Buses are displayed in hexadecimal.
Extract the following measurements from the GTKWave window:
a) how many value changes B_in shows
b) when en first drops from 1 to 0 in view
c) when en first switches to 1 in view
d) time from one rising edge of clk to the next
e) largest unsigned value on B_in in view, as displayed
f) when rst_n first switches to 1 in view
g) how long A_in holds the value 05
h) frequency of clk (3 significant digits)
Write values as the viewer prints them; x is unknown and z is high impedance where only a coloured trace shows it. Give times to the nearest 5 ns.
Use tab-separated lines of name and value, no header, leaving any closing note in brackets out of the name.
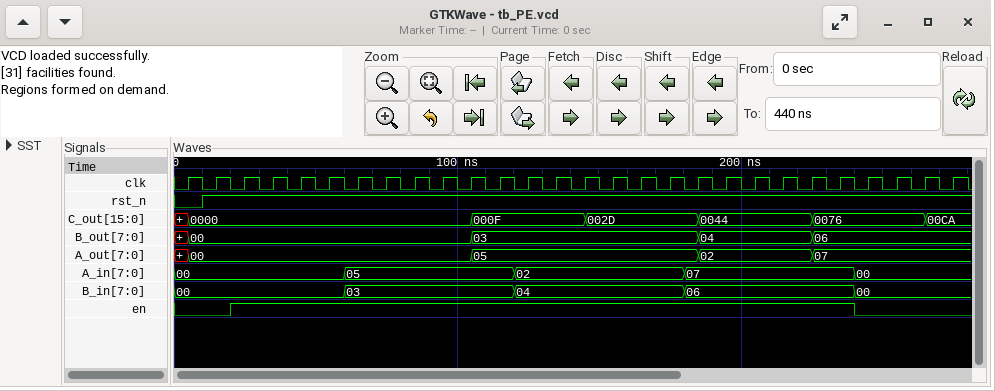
how many value changes B_in shows	4
when en first drops from 1 to 0 in view	240 ns
when en first switches to 1 in view	20 ns
time from one rising edge of clk to the next	10 ns
largest unsigned value on B_in in view, as displayed	06
when rst_n first switches to 1 in view	10 ns
how long A_in holds the value 05	60 ns
frequency of clk	100 MHz
